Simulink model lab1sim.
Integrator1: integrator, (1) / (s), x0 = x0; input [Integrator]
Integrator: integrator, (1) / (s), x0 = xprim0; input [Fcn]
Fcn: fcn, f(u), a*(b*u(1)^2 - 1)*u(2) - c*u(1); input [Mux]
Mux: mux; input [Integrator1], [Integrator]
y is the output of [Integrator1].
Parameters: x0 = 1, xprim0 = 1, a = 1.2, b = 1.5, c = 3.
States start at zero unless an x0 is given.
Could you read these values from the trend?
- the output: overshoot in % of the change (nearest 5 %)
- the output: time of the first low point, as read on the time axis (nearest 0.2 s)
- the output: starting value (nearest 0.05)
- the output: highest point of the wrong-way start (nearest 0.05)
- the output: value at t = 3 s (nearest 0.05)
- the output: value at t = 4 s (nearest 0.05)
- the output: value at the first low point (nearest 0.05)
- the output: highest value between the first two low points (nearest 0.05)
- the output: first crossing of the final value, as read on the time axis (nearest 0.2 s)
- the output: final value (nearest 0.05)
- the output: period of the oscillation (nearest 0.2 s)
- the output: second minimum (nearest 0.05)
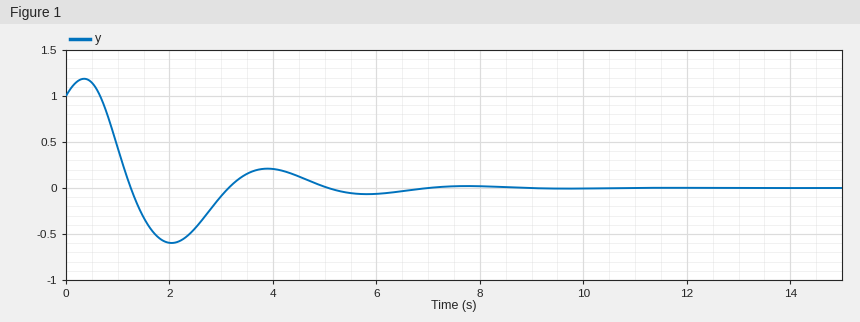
60 %
2.0 s
1.00
1.20
-0.10
0.20
-0.60
0.20
1.2 s
0.00
3.8 s
-0.05
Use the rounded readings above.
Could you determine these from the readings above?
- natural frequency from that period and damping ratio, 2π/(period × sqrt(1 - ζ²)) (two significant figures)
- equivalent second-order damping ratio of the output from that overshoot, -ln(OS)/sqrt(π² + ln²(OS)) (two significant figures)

1.7 rad/s
0.16
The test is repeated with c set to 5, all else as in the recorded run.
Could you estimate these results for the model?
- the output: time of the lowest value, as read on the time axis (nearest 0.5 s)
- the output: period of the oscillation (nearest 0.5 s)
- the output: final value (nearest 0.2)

1.5 s
3.0 s
0.0
